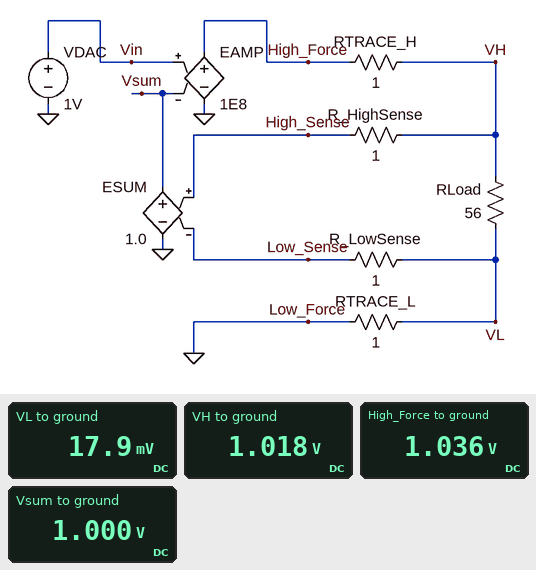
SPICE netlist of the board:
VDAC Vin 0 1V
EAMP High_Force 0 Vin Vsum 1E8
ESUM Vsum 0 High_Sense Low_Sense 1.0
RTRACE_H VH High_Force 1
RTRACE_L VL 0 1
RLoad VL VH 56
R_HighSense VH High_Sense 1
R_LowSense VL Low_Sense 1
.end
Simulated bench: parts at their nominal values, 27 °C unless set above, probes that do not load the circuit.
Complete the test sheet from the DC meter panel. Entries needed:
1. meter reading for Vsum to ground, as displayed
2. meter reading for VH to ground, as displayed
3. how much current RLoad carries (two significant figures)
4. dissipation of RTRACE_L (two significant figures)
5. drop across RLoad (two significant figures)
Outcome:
1.000 V
1.018 V
18 mA
320 µW
1.0 V
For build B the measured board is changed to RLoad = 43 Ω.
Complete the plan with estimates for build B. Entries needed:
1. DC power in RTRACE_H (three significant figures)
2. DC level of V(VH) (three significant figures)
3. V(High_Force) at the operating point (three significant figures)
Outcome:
541 µW
1.02 V
1.05 V
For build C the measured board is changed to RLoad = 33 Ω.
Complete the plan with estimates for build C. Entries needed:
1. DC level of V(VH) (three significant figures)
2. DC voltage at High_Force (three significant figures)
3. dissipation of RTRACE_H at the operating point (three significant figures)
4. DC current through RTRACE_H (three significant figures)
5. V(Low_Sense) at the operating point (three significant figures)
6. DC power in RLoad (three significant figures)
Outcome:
1.03 V
1.06 V
918 µW
30.3 mA
30.3 mV
30.3 mW
